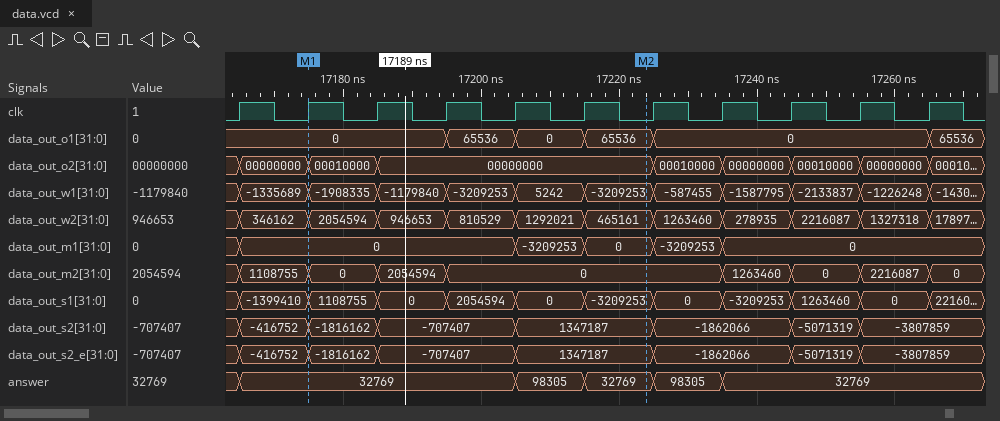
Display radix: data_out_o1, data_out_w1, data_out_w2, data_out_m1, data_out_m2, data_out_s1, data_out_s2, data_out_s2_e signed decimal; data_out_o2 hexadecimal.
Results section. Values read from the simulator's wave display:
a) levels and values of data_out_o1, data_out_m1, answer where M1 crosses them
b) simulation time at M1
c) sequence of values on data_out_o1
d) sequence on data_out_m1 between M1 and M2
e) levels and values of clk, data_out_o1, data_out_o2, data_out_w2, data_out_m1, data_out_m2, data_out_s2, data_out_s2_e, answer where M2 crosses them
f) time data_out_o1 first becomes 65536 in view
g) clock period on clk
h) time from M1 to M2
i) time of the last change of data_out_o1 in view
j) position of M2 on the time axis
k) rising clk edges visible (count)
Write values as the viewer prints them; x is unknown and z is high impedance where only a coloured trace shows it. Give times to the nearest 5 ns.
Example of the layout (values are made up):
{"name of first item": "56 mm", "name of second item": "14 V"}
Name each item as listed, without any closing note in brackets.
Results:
{"levels and values of data_out_o1, data_out_m1, answer where M1 crosses them": "data_out_o1=0, data_out_m1=0, answer=32769", "simulation time at M1": "17175 ns", "sequence of values on data_out_o1": "0, 65536, 0, 65536, 0, 65536", "sequence on data_out_m1 between M1 and M2": "0, -3209253, 0", "levels and values of clk, data_out_o1, data_out_o2, data_out_w2, data_out_m1, data_out_m2, data_out_s2, data_out_s2_e, answer where M2 crosses them": "clk=0, data_out_o1=65536, data_out_o2=00000000, data_out_w2=465161, data_out_m1=0, data_out_m2=0, data_out_s2=1347187, data_out_s2_e=1347187, answer=32769", "time data_out_o1 first becomes 65536 in view": "17195 ns", "clock period on clk": "10 ns", "time from M1 to M2": "50 ns", "time of the last change of data_out_o1 in view": "17265 ns", "position of M2 on the time axis": "17225 ns", "rising clk edges visible": "11"}
